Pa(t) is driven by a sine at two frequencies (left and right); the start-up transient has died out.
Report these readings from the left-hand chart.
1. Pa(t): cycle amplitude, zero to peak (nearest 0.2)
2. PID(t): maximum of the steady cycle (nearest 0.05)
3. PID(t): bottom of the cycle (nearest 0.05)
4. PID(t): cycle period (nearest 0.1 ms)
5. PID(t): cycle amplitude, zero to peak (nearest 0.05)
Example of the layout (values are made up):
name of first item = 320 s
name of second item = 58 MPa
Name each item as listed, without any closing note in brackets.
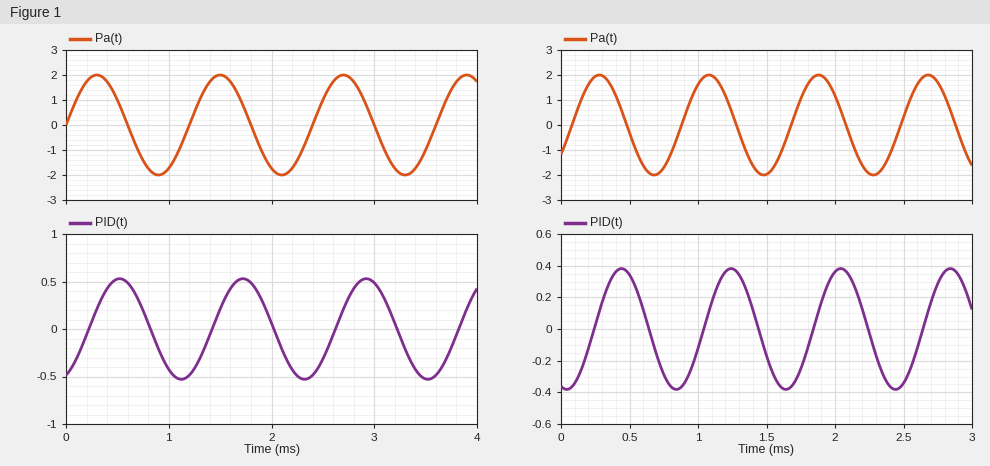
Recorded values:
Pa(t): cycle amplitude, zero to peak = 2.0
PID(t): maximum of the steady cycle = 0.55
PID(t): bottom of the cycle = -0.55
PID(t): cycle period = 1.2 ms
PID(t): cycle amplitude, zero to peak = 0.55
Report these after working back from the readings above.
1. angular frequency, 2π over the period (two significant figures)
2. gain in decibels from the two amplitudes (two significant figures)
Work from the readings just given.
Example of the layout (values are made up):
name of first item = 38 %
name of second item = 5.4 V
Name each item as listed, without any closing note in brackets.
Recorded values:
angular frequency, 2π over the period = 5.2 rad/ms
gain in decibels from the two amplitudes = -11 dB
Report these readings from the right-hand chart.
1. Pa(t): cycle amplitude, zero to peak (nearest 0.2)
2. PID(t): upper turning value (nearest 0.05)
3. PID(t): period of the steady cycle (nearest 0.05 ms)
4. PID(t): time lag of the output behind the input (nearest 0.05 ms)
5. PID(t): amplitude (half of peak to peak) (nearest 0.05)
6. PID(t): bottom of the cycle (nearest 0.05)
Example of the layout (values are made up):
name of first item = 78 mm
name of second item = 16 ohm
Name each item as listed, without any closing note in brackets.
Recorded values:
Pa(t): cycle amplitude, zero to peak = 2.0
PID(t): upper turning value = 0.40
PID(t): period of the steady cycle = 0.80 ms
PID(t): time lag of the output behind the input = 0.15 ms
PID(t): amplitude (half of peak to peak) = 0.40
PID(t): bottom of the cycle = -0.40
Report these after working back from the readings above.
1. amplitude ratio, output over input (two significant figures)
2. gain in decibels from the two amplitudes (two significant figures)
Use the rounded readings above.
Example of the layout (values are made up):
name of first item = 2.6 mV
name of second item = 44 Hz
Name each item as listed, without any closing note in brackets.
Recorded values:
amplitude ratio, output over input = 0.20
gain in decibels from the two amplitudes = -14 dB
